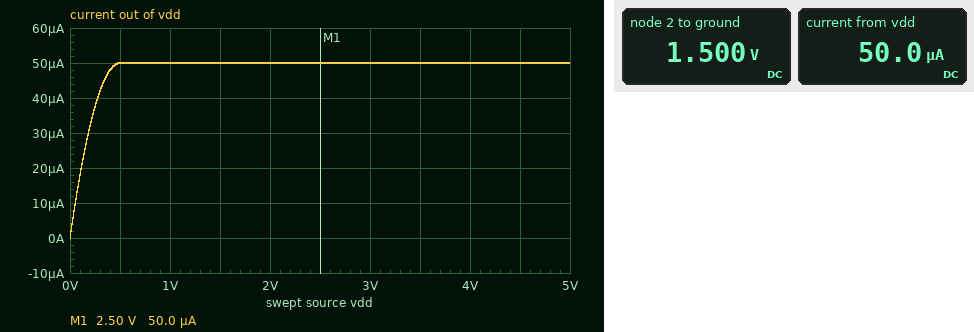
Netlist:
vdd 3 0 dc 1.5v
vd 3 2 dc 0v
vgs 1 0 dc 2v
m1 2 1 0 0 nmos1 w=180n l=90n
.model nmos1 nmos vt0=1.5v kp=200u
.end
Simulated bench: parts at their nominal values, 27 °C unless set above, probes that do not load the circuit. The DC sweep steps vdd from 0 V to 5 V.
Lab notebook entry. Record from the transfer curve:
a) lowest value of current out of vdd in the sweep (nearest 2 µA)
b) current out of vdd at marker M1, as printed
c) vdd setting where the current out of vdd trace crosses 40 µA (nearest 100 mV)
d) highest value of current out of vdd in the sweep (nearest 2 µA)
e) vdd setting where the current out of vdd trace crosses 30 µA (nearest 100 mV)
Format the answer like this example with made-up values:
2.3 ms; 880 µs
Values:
0 A; 50.0 µA; 300 mV; 50 µA; 200 mV
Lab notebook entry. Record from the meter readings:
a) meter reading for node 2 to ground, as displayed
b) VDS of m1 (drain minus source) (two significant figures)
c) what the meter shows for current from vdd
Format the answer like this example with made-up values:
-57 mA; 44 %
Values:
1.500 V; 1.5 V; 50.0 µA
